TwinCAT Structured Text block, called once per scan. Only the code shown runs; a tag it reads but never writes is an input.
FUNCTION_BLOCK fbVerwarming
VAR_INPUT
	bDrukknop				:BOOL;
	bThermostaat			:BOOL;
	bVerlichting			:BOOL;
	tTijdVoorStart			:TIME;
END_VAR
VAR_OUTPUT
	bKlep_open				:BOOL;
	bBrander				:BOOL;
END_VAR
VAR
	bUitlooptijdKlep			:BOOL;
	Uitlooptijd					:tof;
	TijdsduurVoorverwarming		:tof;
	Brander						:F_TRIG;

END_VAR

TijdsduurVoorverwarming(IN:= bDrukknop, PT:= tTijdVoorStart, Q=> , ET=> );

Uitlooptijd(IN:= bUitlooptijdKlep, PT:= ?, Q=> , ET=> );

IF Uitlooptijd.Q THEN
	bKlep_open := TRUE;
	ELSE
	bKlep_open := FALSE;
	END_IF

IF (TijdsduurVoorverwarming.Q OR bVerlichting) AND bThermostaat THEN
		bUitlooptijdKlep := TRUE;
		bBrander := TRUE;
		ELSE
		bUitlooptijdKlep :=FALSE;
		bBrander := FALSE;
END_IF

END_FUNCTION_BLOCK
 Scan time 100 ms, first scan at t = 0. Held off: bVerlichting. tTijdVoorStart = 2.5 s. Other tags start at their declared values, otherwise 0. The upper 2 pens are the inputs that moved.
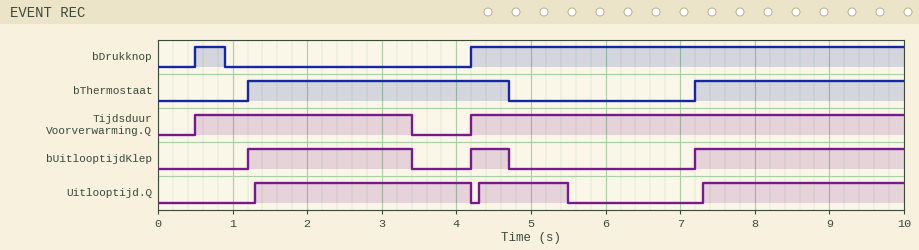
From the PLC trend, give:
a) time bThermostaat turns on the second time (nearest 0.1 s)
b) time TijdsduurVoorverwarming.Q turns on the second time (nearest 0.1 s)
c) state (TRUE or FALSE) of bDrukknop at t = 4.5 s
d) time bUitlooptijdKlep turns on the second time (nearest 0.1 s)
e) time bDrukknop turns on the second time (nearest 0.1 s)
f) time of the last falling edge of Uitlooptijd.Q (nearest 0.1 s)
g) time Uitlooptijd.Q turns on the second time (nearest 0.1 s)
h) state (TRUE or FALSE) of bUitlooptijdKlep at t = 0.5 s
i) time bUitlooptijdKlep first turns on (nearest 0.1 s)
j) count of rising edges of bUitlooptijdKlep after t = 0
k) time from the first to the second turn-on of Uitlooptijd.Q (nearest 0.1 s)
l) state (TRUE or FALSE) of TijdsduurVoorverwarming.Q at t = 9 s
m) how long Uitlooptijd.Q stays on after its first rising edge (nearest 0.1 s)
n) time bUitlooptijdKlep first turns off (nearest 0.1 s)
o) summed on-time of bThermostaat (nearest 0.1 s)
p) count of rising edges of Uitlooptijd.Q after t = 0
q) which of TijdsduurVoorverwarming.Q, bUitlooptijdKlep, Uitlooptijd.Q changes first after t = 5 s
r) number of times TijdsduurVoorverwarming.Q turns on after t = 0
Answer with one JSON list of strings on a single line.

["7.2 s", "4.2 s", "TRUE", "4.2 s", "4.2 s", "5.5 s", "4.3 s", "FALSE", "1.2 s", "3", "3.0 s", "TRUE", "2.9 s", "3.4 s", "6.3 s", "3", "Uitlooptijd.Q", "2"]
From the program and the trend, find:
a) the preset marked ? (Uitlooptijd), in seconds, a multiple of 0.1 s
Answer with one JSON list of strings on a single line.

["0.7 s"]
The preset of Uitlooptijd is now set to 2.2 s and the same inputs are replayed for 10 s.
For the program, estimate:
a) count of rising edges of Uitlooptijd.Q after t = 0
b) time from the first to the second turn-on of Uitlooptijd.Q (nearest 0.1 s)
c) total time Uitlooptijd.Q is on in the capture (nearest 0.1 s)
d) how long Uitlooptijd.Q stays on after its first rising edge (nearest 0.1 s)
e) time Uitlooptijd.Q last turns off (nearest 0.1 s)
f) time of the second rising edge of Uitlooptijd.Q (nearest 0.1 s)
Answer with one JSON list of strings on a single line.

["2", "6.0 s", "8.4 s", "5.7 s", "7.0 s", "7.3 s"]
